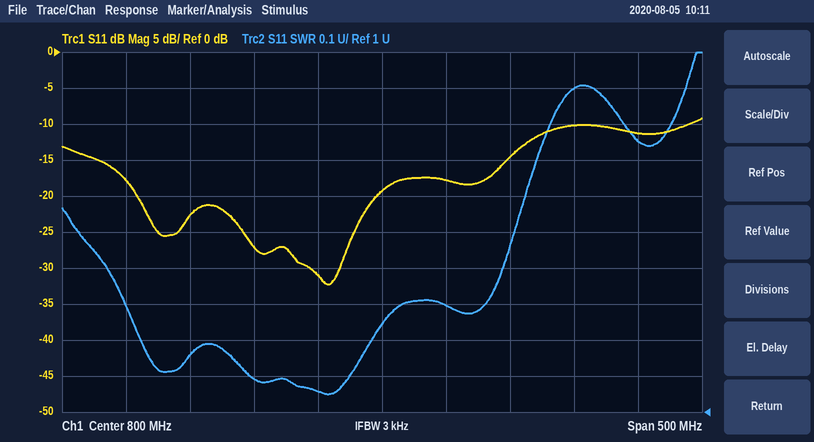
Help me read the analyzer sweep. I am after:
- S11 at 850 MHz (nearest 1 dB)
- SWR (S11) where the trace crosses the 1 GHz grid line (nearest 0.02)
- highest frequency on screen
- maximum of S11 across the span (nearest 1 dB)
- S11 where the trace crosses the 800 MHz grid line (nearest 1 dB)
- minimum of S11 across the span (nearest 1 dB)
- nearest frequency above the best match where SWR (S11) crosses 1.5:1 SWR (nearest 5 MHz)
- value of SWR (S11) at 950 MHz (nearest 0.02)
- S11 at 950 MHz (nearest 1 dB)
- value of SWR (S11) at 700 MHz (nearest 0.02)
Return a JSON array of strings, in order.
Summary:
["-18 dB", "1.76", "1.05 GHz", "-9 dB", "-19 dB", "-32 dB", "905 MHz", "1.90", "-10 dB", "1.10"]
